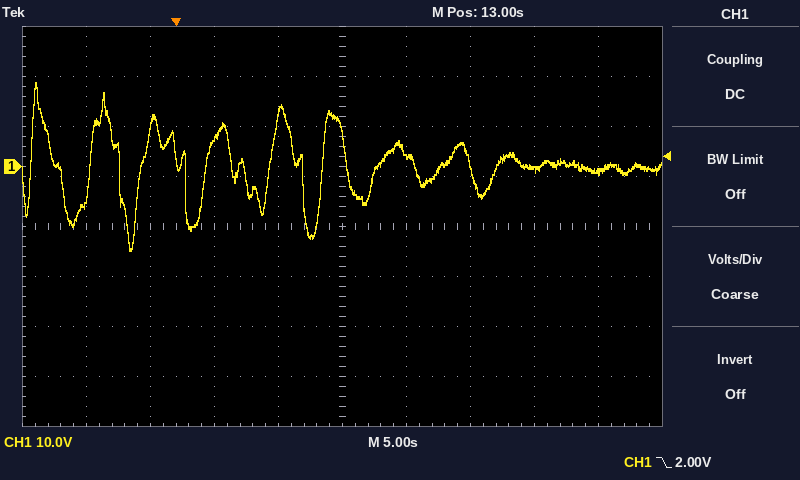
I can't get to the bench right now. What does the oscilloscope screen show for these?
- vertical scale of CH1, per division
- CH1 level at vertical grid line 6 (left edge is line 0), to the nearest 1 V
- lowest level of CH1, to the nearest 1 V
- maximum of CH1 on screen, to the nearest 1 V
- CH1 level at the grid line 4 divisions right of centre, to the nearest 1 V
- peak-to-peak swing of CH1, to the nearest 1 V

10 V
2 V
-17 V
17 V
-1 V
34 V
